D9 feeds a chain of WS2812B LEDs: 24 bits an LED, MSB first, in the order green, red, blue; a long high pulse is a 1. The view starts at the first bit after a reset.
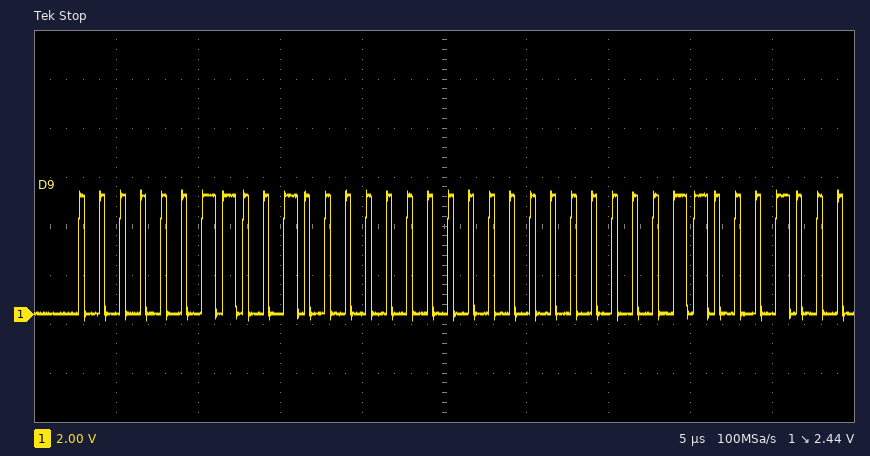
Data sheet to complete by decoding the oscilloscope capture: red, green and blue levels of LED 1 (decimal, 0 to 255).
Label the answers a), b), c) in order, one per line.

a) 32, 3, 0
